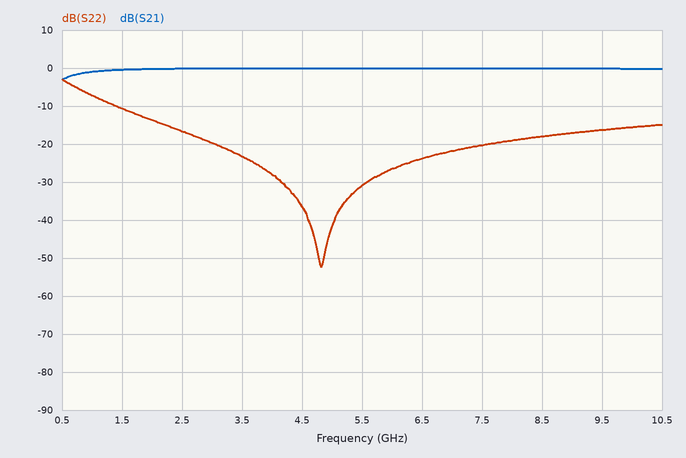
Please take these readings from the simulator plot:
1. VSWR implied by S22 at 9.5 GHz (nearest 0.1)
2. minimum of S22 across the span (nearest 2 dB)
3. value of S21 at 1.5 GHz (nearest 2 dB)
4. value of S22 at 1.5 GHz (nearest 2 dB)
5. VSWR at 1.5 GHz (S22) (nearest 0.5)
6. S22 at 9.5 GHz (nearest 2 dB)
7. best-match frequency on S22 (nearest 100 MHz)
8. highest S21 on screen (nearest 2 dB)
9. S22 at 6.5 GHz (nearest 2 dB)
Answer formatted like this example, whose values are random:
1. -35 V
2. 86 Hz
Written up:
1. 1.4
2. -52 dB
3. 0 dB
4. -10 dB
5. 2.0
6. -16 dB
7. 4.8 GHz
8. 0 dB
9. -24 dB
